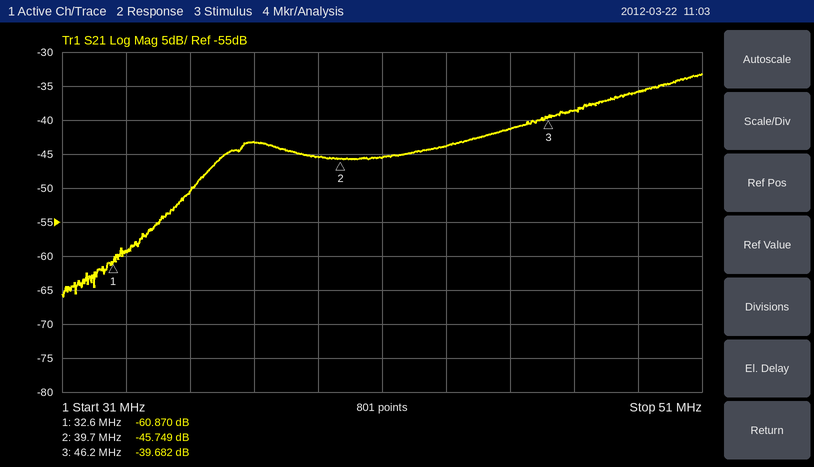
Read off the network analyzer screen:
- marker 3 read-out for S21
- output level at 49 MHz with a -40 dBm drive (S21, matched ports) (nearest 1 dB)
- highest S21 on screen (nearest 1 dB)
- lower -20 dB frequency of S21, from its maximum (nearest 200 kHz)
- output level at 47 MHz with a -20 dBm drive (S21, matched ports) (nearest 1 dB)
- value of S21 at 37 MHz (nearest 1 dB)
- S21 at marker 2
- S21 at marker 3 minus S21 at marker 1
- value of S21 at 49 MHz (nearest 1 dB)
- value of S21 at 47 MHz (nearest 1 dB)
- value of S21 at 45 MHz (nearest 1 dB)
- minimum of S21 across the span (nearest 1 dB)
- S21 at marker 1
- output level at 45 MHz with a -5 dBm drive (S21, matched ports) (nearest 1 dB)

-39.682 dB
-76 dBm
-33 dB
34.4 MHz
-59 dBm
-43 dB
-45.749 dB
21.188 dB
-36 dB
-39 dB
-41 dB
-66 dB
-60.870 dB
-46 dBm
